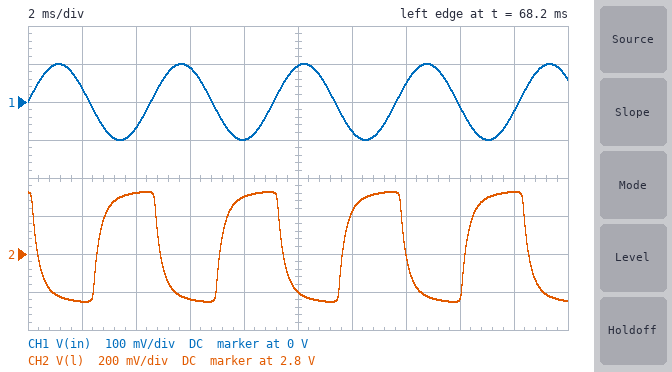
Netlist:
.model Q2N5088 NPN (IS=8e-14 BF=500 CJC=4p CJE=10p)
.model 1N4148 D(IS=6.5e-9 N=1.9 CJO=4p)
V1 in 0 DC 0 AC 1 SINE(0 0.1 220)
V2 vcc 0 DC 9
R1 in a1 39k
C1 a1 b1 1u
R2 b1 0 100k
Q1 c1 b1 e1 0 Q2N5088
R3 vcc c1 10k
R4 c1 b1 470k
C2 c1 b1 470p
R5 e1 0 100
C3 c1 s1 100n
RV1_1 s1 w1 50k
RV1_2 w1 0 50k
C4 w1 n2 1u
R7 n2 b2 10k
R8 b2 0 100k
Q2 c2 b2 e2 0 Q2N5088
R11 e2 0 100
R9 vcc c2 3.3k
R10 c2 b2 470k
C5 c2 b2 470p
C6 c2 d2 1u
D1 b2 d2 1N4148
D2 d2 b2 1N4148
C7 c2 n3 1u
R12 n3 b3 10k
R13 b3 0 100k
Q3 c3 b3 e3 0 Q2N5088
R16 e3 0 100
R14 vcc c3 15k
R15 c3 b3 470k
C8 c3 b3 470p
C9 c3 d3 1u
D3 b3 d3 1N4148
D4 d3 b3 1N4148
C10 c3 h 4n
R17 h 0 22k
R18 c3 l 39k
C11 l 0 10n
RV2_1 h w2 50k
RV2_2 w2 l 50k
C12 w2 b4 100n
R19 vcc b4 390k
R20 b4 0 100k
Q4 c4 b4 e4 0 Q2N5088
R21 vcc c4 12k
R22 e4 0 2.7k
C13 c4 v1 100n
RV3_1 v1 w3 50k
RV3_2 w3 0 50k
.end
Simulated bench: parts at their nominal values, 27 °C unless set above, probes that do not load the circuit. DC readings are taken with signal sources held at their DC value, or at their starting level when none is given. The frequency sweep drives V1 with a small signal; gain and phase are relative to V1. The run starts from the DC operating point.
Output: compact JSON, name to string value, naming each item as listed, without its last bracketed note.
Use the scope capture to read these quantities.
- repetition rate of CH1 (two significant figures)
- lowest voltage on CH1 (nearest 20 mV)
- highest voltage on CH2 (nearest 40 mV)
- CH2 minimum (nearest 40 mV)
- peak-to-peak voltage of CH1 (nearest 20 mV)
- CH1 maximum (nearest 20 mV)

{"repetition rate of CH1": "220 Hz", "lowest voltage on CH1": "-100 mV", "highest voltage on CH2": "3.12 V", "CH2 minimum": "2.56 V", "peak-to-peak voltage of CH1": "200 mV", "CH1 maximum": "100 mV"}
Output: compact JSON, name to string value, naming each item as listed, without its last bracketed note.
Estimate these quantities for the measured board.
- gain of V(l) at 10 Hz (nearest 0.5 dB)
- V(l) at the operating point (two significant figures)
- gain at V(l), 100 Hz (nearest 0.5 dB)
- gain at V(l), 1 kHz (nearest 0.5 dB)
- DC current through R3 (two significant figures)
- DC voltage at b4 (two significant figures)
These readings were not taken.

{"gain of V(l) at 10 Hz": "40.5 dB", "V(l) at the operating point": "2.8 V", "gain at V(l), 100 Hz": "51.5 dB", "gain at V(l), 1 kHz": "39.0 dB", "DC current through R3": "490 µA", "DC voltage at b4": "1.8 V"}
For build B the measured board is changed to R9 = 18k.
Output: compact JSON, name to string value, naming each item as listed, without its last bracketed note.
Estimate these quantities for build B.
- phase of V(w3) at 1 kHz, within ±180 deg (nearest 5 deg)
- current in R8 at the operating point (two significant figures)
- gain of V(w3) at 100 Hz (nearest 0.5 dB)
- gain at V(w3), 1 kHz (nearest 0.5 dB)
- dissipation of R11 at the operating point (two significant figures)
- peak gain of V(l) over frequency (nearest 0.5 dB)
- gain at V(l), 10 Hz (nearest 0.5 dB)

{"phase of V(w3) at 1 kHz, within ±180 deg": "-120 deg", "current in R8 at the operating point": "6.0 µA", "gain of V(w3) at 100 Hz": "52.5 dB", "gain at V(w3), 1 kHz": "38.5 dB", "dissipation of R11 at the operating point": "8.4 µW", "peak gain of V(l) over frequency": "54.5 dB", "gain at V(l), 10 Hz": "43.5 dB"}
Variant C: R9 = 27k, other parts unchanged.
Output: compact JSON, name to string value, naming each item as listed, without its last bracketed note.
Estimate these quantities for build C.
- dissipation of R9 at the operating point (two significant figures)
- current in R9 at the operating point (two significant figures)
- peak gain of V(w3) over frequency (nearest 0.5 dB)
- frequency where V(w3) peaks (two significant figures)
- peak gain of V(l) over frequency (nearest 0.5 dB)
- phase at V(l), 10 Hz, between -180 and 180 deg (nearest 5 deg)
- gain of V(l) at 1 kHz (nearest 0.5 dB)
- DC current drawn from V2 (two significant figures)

{"dissipation of R9 at the operating point": "1.1 mW", "current in R9 at the operating point": "200 µA", "peak gain of V(w3) over frequency": "52.5 dB", "frequency where V(w3) peaks": "110 Hz", "peak gain of V(l) over frequency": "54.5 dB", "phase at V(l), 10 Hz, between -180 and 180 deg": "-45 deg", "gain of V(l) at 1 kHz": "40.5 dB", "DC current drawn from V2": "1.5 mA"}
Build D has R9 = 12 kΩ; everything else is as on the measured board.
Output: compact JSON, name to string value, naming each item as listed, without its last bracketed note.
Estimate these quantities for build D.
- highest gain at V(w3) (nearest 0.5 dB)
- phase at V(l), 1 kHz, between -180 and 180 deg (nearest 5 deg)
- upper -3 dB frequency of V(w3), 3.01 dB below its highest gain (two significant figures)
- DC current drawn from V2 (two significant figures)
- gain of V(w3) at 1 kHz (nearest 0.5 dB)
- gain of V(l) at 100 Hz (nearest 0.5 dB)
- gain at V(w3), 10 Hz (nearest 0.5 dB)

{"highest gain at V(w3)": "52.0 dB", "phase at V(l), 1 kHz, between -180 and 180 deg": "5 deg", "upper -3 dB frequency of V(w3), 3.01 dB below its highest gain": "370 Hz", "DC current drawn from V2": "1.7 mA", "gain of V(w3) at 1 kHz": "38.0 dB", "gain of V(l) at 100 Hz": "54.0 dB", "gain at V(w3), 10 Hz": "31.5 dB"}
